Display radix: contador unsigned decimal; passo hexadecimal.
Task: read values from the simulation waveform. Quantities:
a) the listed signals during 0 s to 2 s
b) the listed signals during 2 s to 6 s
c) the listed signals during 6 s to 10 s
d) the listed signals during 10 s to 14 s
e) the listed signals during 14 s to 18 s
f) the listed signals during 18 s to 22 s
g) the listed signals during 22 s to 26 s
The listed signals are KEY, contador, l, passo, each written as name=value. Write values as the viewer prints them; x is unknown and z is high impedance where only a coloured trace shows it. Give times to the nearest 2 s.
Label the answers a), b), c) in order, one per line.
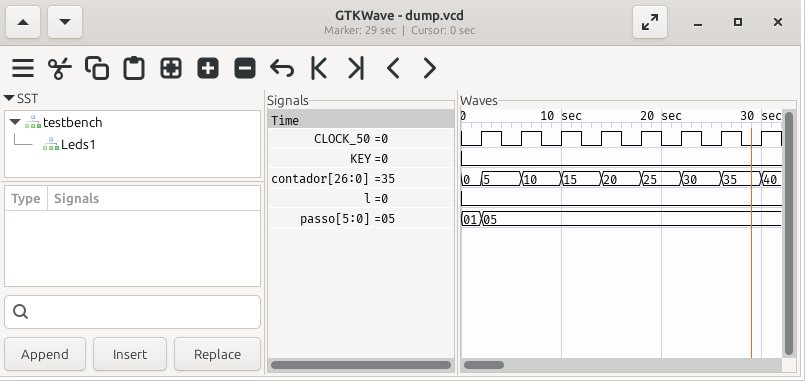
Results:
a) KEY=0, contador=0, l=0, passo=01
b) KEY=0, contador=5, l=0, passo=05
c) KEY=0, contador=10, l=0, passo=05
d) KEY=0, contador=15, l=0, passo=05
e) KEY=0, contador=20, l=0, passo=05
f) KEY=0, contador=25, l=0, passo=05
g) KEY=0, contador=30, l=0, passo=05
